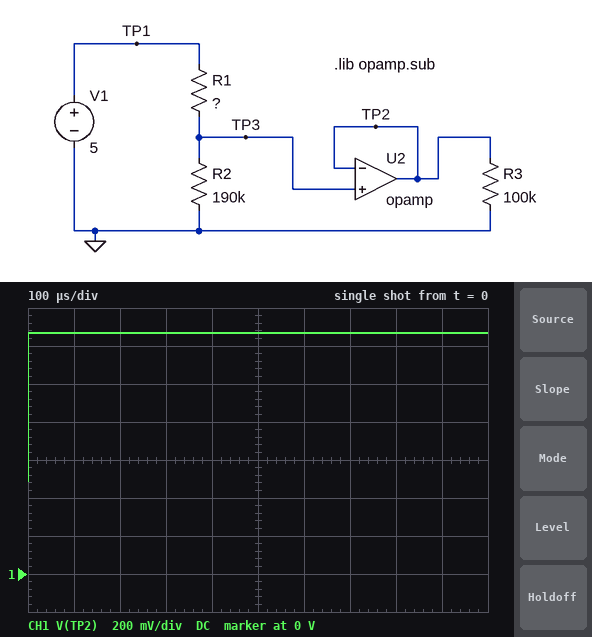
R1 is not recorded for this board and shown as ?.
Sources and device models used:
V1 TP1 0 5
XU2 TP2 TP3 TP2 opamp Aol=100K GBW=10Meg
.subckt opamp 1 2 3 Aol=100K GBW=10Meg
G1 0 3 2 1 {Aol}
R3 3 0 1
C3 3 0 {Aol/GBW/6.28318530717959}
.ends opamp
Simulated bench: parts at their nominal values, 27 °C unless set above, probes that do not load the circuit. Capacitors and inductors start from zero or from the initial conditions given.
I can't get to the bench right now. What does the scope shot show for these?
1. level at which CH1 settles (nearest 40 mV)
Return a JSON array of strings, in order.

["1.28 V"]
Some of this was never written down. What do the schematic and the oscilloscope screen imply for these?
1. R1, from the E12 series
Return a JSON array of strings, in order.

["560 kΩ"]
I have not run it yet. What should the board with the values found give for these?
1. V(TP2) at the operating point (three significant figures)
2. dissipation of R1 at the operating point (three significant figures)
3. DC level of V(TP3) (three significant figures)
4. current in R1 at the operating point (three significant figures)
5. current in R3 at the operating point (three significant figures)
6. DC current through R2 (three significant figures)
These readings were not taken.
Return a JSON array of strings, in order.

["1.27 V", "24.9 µW", "1.27 V", "6.67 µA", "12.7 µA", "6.67 µA"]
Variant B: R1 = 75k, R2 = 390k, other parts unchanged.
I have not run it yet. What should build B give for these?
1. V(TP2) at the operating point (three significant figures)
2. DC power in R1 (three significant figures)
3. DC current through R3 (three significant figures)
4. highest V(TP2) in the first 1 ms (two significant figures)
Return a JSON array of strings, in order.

["4.19 V", "8.67 µW", "41.9 µA", "4.2 V"]
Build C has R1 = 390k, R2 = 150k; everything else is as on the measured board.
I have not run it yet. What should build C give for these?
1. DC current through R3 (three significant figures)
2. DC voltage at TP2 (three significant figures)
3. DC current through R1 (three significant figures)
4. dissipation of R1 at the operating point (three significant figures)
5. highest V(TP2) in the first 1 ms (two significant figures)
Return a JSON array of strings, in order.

["13.9 µA", "1.39 V", "9.26 µA", "33.4 µW", "1.4 V"]
